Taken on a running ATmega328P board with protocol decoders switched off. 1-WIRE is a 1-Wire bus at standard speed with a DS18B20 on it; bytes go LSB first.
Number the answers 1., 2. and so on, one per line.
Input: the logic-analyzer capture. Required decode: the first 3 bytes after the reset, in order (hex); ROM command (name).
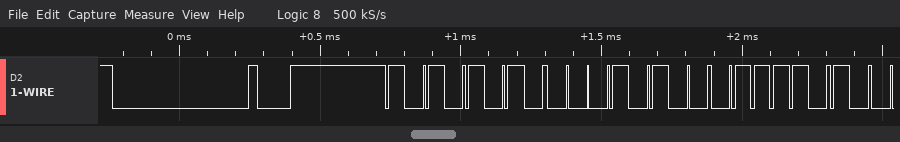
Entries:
1. 55 28 5E
2. Match ROM
